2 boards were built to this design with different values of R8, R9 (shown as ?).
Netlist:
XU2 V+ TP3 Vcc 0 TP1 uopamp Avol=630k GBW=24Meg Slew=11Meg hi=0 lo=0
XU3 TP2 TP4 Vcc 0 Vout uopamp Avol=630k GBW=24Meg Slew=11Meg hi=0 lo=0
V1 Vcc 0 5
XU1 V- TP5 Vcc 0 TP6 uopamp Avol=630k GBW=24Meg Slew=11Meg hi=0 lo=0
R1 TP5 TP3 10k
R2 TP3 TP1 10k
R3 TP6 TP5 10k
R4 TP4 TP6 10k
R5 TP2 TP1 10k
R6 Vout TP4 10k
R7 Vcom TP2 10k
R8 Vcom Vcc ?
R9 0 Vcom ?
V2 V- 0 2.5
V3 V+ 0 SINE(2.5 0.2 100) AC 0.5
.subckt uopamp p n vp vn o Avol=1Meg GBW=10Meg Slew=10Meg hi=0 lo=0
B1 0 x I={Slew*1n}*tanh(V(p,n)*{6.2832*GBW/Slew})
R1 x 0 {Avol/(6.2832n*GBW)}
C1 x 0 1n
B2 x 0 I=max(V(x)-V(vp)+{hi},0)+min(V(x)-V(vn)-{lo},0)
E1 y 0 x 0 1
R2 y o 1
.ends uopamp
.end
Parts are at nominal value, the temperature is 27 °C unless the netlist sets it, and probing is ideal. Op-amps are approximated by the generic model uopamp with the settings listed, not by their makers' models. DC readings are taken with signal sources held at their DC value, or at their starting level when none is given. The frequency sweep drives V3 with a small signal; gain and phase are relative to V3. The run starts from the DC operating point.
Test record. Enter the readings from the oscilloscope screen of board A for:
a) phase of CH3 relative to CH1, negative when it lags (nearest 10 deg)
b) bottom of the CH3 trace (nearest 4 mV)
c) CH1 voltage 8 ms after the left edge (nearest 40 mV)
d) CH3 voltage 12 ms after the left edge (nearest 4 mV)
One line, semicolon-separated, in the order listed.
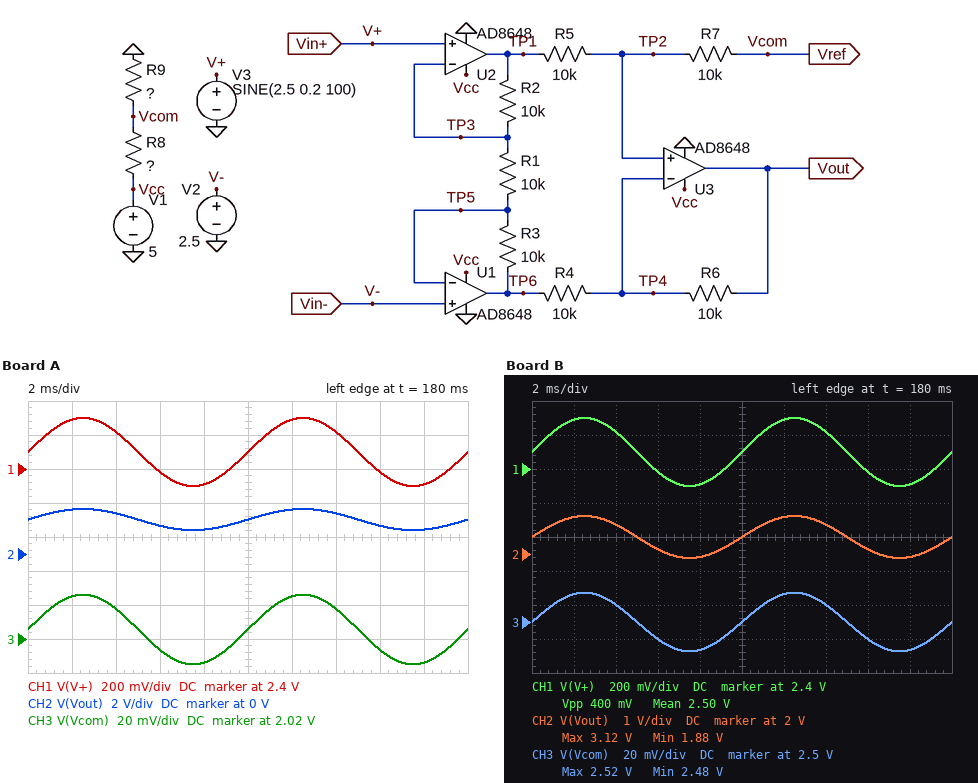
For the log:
0 deg; 2.004 V; 2.32 V; 2.044 V
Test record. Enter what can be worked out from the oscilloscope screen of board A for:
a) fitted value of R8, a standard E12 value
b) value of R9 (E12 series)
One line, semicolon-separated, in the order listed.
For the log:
2.7 kΩ; 1.8 kΩ
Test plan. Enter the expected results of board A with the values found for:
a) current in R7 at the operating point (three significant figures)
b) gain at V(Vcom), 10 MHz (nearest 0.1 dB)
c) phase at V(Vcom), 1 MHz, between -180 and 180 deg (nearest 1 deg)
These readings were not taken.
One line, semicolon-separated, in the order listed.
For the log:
23.7 µA; -23.1 dB; -6 deg
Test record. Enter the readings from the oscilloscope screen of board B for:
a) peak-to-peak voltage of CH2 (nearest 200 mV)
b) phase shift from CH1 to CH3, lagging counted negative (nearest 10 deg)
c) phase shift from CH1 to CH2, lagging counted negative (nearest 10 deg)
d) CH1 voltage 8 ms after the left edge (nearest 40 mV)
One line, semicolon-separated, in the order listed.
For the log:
1.2 V; 0 deg; 0 deg; 2.32 V
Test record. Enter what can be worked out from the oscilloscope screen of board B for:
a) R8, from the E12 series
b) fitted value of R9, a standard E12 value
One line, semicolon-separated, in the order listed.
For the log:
1.8 kΩ; 1.8 kΩ
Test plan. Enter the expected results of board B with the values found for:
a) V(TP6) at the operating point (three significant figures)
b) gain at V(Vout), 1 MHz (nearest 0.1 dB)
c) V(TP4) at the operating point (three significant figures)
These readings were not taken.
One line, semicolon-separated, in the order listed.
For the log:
2.50 V; 9.7 dB; 2.50 V
